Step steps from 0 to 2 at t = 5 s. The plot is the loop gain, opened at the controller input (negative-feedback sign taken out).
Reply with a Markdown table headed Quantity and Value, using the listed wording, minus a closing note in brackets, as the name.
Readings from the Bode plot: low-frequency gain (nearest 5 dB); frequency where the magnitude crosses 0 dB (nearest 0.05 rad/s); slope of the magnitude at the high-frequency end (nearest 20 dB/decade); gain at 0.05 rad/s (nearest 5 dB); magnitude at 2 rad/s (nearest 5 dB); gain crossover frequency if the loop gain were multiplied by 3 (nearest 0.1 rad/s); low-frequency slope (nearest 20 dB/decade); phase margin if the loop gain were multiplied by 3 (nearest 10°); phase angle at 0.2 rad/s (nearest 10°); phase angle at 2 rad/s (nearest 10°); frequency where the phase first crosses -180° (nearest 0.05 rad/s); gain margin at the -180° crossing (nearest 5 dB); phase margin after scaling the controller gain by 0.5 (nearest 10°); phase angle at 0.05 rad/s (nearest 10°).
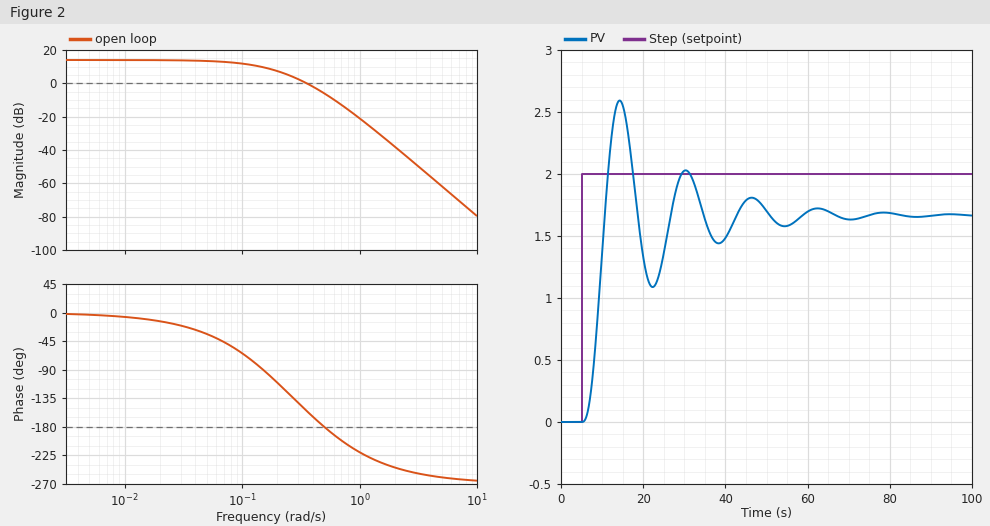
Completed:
| Quantity | Value |
|---|---|
| low-frequency gain | 15 dB |
| frequency where the magnitude crosses 0 dB | 0.35 rad/s |
| slope of the magnitude at the high-frequency end | -60 dB/decade |
| gain at 0.05 rad/s | 15 dB |
| magnitude at 2 rad/s | -40 dB |
| gain crossover frequency if the loop gain were multiplied by 3 | 0.6 rad/s |
| low-frequency slope | 0 dB/decade |
| phase margin if the loop gain were multiplied by 3 | -10° |
| phase angle at 0.2 rad/s | -110° |
| phase angle at 2 rad/s | -240° |
| frequency where the phase first crosses -180° | 0.50 rad/s |
| gain margin at the -180° crossing | 5 dB |
| phase margin after scaling the controller gain by 0.5 | 60° |
| phase angle at 0.05 rad/s | -30° |
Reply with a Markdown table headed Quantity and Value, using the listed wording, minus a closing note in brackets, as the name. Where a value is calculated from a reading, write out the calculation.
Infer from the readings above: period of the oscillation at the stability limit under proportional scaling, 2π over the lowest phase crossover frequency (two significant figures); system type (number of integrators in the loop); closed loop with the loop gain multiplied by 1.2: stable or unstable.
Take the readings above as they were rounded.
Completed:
| Quantity | Value |
|---|---|
| period of the oscillation at the stability limit under proportional scaling, 2π over the lowest phase crossover frequency | 2π / 0.5 = 13 s |
| system type | 0 |
| closed loop with the loop gain multiplied by 1.2: stable or unstable | stable |
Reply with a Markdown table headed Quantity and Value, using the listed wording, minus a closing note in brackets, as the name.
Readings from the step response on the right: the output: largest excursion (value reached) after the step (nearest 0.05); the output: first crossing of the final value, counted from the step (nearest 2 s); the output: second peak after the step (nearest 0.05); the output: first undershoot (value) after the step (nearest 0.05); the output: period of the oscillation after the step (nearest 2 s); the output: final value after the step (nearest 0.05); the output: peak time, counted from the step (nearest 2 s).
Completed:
| Quantity | Value |
|---|---|
| the output: largest excursion (value reached) after the step | 2.60 |
| the output: first crossing of the final value, counted from the step | 6 s |
| the output: second peak after the step | 2.05 |
| the output: first undershoot (value) after the step | 1.10 |
| the output: period of the oscillation after the step | 16 s |
| the output: final value after the step | 1.65 |
| the output: peak time, counted from the step | 10 s |
